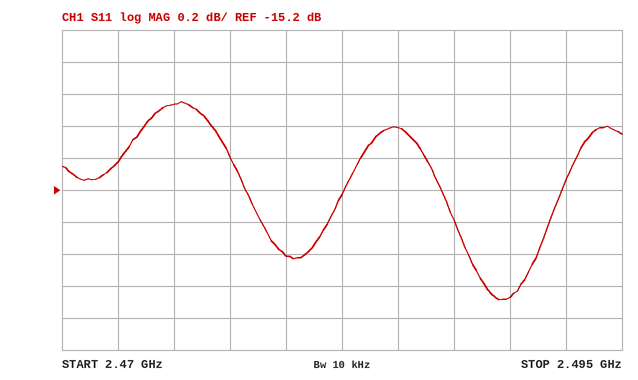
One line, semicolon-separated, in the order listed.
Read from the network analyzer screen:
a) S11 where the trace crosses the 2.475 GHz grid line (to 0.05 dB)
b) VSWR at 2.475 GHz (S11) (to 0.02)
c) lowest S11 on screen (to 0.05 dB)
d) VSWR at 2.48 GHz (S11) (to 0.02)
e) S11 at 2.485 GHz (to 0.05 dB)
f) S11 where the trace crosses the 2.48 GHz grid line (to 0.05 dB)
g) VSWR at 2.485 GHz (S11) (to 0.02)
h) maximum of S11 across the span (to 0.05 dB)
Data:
-14.65 dB; 1.46; -15.90 dB; 1.40; -14.80 dB; -15.60 dB; 1.44; -14.65 dB
